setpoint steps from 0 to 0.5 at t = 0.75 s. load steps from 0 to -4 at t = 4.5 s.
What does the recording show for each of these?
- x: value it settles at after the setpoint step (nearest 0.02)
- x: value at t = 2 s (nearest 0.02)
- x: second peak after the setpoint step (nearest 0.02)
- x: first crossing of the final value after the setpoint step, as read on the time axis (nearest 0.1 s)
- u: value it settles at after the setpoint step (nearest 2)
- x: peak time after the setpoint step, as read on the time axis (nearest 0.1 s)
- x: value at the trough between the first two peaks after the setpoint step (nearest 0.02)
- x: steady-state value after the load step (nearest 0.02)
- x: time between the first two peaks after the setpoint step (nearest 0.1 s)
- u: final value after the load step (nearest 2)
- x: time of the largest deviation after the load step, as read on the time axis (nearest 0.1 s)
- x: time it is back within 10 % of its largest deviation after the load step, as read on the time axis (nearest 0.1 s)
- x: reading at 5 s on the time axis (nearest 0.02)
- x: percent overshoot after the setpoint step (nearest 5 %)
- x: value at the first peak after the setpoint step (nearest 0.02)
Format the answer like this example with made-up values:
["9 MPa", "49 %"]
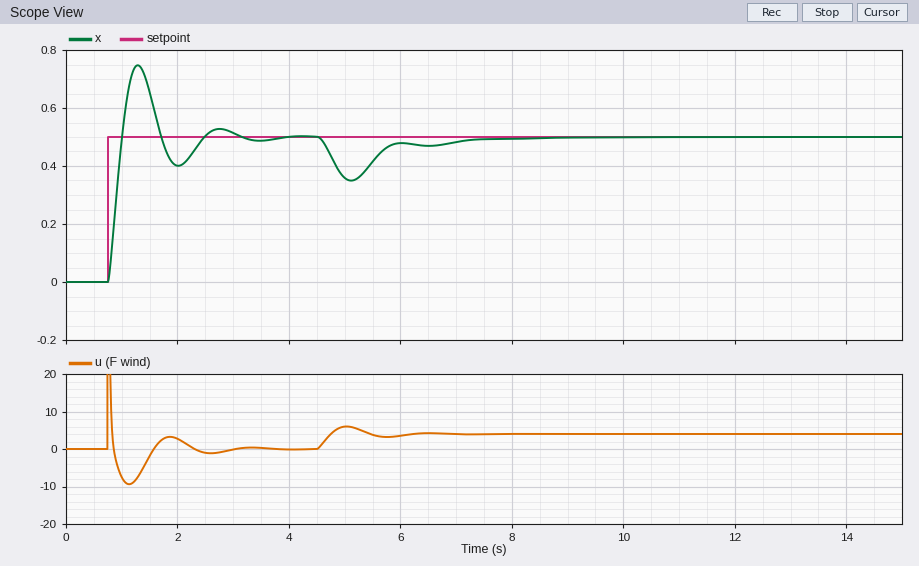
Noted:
["0.50", "0.40", "0.52", "1.0 s", "0", "1.3 s", "0.40", "0.50", "1.5 s", "4", "5.1 s", "7.1 s", "0.36", "50 %", "0.74"]
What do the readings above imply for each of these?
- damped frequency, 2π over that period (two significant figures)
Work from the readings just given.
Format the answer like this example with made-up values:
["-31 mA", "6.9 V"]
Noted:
["4.2 rad/s"]
